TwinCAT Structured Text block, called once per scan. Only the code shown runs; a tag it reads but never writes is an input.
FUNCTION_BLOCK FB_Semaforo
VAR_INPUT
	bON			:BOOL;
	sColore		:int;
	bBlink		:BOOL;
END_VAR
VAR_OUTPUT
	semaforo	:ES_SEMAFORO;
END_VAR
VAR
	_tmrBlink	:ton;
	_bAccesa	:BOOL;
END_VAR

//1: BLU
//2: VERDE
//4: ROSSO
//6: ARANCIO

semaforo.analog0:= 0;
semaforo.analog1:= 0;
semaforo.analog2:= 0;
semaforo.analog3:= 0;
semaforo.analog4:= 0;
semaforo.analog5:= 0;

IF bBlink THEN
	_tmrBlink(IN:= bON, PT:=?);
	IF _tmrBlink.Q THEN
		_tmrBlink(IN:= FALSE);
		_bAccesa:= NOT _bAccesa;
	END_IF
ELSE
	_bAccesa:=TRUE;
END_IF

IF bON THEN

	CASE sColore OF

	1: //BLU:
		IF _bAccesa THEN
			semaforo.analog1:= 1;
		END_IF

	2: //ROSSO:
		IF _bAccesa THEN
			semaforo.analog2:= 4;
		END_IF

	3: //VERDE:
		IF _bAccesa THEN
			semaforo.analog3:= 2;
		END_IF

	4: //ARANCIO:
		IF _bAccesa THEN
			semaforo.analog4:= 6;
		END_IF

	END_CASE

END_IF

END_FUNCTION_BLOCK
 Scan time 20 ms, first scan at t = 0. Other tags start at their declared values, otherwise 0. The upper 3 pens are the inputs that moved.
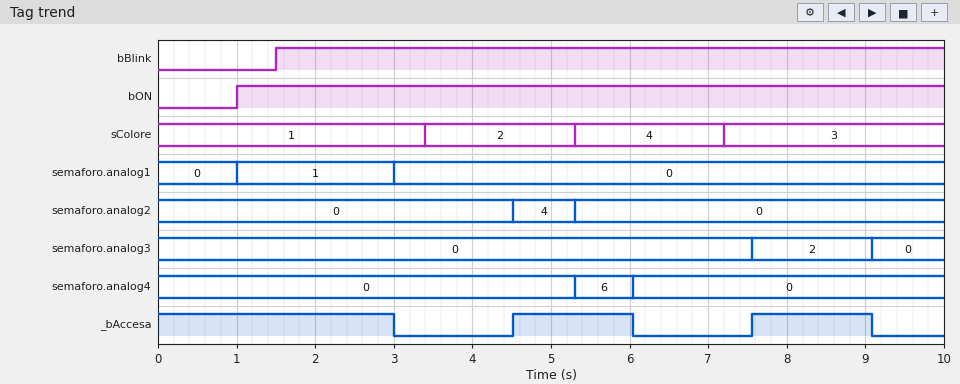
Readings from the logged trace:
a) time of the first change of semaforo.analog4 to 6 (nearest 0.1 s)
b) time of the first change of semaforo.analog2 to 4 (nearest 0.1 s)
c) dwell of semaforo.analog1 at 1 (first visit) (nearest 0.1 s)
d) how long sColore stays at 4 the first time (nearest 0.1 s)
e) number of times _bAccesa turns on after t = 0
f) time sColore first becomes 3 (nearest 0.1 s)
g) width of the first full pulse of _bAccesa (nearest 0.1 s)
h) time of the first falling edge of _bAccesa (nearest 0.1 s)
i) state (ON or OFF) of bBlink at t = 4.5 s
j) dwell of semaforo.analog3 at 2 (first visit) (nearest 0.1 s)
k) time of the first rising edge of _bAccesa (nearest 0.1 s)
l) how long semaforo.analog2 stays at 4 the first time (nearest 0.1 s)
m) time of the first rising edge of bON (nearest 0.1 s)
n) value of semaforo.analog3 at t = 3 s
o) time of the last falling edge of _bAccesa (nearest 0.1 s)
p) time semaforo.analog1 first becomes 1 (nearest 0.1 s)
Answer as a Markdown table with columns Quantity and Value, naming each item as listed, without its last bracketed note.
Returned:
| Quantity | Value |
|---|---|
| time of the first change of semaforo.analog4 to 6 | 5.3 s |
| time of the first change of semaforo.analog2 to 4 | 4.5 s |
| dwell of semaforo.analog1 at 1 (first visit) | 2.0 s |
| how long sColore stays at 4 the first time | 1.9 s |
| number of times _bAccesa turns on after t = 0 | 2 |
| time sColore first becomes 3 | 7.2 s |
| width of the first full pulse of _bAccesa | 1.5 s |
| time of the first falling edge of _bAccesa | 3.0 s |
| state (ON or OFF) of bBlink at t = 4.5 s | ON |
| dwell of semaforo.analog3 at 2 (first visit) | 1.5 s |
| time of the first rising edge of _bAccesa | 4.5 s |
| how long semaforo.analog2 stays at 4 the first time | 0.8 s |
| time of the first rising edge of bON | 1.0 s |
| value of semaforo.analog3 at t = 3 s | 0 |
| time of the last falling edge of _bAccesa | 9.1 s |
| time semaforo.analog1 first becomes 1 | 1.0 s |
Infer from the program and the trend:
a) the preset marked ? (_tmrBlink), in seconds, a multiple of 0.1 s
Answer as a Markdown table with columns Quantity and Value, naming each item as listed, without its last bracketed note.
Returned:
| Quantity | Value |
|---|---|
| the preset marked ? (_tmrBlink), in seconds, a multiple of 0.1 s | 1.5 s |
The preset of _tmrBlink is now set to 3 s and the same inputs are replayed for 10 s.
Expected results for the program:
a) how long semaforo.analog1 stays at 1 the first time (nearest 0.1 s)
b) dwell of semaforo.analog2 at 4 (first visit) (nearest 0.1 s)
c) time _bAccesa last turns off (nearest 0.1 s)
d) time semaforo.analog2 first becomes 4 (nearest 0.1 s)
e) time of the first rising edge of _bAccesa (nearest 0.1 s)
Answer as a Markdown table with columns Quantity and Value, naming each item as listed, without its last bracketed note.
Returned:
| Quantity | Value |
|---|---|
| how long semaforo.analog1 stays at 1 the first time | 2.4 s |
| dwell of semaforo.analog2 at 4 (first visit) | 1.1 s |
| time _bAccesa last turns off | 4.5 s |
| time semaforo.analog2 first becomes 4 | 3.4 s |
| time of the first rising edge of _bAccesa | 7.5 s |
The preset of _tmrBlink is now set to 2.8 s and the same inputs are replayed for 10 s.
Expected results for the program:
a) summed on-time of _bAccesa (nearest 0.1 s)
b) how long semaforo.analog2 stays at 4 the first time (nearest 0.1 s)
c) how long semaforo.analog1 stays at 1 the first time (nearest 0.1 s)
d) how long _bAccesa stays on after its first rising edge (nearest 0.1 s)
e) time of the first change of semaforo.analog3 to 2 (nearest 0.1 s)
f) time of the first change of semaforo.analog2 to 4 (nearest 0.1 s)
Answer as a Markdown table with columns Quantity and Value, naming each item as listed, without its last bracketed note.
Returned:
| Quantity | Value |
|---|---|
| summed on-time of _bAccesa | 7.1 s |
| how long semaforo.analog2 stays at 4 the first time | 0.9 s |
| how long semaforo.analog1 stays at 1 the first time | 2.4 s |
| how long _bAccesa stays on after its first rising edge | 2.8 s |
| time of the first change of semaforo.analog3 to 2 | 7.2 s |
| time of the first change of semaforo.analog2 to 4 | 3.4 s |
